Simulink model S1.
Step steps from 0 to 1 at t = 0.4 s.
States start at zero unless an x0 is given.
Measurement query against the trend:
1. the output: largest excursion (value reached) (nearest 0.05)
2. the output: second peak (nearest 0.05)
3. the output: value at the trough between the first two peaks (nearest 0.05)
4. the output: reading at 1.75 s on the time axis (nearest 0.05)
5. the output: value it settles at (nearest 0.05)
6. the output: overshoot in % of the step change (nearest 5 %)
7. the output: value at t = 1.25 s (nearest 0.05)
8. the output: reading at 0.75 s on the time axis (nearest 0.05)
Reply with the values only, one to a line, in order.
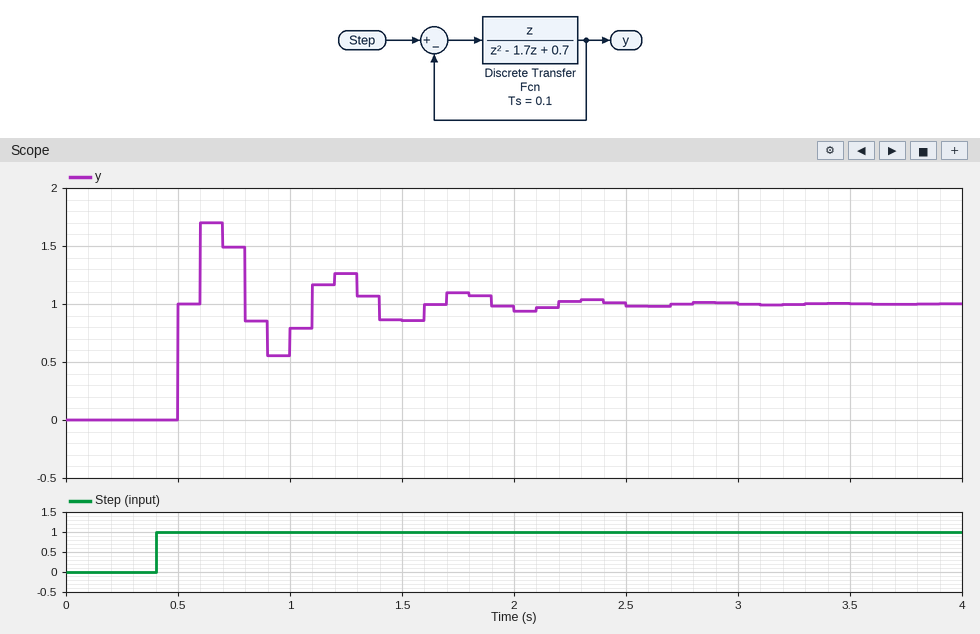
1.70
1.25
0.55
1.10
1.00
70 %
1.25
1.50
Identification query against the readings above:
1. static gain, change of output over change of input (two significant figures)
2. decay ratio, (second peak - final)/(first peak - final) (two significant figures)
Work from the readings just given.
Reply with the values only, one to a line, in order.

1.0
0.36
